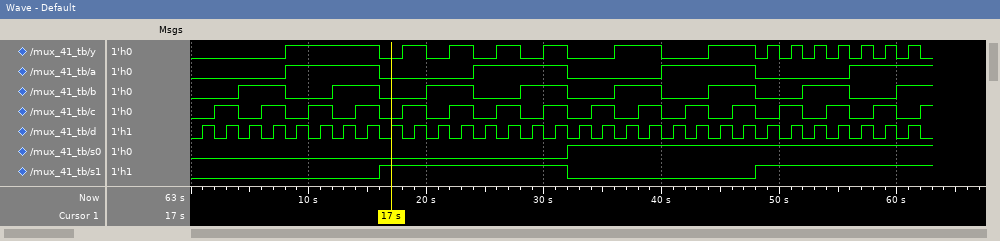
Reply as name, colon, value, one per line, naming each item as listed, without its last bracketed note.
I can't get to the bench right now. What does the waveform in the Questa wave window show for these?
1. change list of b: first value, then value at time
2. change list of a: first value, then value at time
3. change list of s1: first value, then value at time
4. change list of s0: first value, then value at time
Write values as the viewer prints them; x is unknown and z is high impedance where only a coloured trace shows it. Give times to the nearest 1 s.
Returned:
change list of b: first value, then value at time: 0, 1 at 4 s, 0 at 8 s, 1 at 12 s, 0 at 16 s, 1 at 20 s, 0 at 24 s, 1 at 28 s, 0 at 32 s, 1 at 36 s, 0 at 40 s, 1 at 44 s, 0 at 48 s, 1 at 52 s, 0 at 56 s, 1 at 60 s
change list of a: first value, then value at time: 0, 1 at 8 s, 0 at 16 s, 1 at 24 s, 0 at 32 s, 1 at 40 s, 0 at 48 s, 1 at 56 s
change list of s1: first value, then value at time: 0, 1 at 16 s, 0 at 32 s, 1 at 48 s
change list of s0: first value, then value at time: 0, 1 at 32 s
